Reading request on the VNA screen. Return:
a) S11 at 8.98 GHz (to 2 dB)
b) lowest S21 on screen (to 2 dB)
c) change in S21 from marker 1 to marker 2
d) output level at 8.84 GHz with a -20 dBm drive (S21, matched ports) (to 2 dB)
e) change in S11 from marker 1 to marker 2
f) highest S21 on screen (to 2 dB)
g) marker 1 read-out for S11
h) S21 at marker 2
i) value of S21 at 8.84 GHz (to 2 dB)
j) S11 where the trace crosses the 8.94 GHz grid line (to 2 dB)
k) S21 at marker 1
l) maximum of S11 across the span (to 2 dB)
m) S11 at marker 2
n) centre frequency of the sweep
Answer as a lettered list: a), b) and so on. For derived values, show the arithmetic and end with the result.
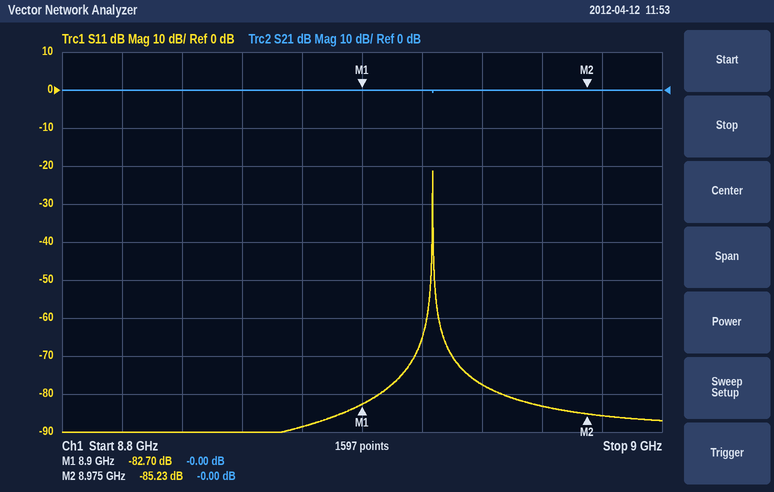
a) -86 dB
b) 0 dB
c) -0 − (-0) = 0.00 dB
d) -20 dBm + (0 dB) = -20 dBm
e) -85.23 − (-82.7) = -2.53 dB
f) 0 dB
g) -82.70 dB
h) -0.00 dB
i) 0 dB
j) -78 dB
k) -0.00 dB
l) -22 dB
m) -85.23 dB
n) 8.9 GHz
